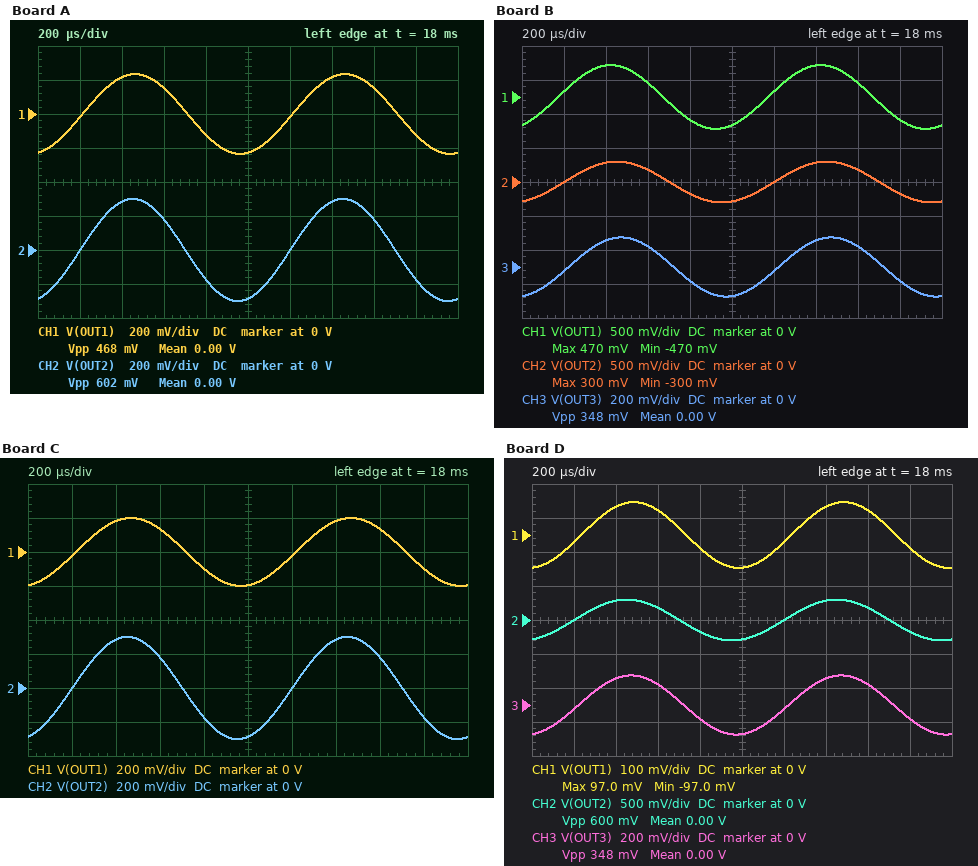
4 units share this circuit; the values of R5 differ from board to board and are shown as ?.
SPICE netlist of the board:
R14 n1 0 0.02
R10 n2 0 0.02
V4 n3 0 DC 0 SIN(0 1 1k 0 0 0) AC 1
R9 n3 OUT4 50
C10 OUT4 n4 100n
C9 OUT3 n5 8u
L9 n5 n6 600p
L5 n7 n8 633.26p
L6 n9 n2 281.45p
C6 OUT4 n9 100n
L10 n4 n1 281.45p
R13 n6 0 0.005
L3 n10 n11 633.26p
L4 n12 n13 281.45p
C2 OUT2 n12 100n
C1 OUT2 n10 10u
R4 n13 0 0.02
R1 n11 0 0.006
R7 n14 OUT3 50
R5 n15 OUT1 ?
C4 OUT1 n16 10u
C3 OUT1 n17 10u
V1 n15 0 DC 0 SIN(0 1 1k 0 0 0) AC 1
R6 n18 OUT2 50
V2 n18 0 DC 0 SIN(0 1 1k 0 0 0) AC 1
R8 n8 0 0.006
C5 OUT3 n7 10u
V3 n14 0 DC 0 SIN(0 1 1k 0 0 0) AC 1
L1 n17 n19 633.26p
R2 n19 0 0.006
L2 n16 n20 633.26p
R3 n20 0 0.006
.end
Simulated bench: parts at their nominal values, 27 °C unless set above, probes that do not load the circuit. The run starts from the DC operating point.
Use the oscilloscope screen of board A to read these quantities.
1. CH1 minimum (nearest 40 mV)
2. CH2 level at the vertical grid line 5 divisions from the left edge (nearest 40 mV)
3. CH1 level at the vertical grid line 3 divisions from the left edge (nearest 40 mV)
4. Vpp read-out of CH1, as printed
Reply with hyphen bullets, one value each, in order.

- -240 mV
- -280 mV
- 160 mV
- 468 mV
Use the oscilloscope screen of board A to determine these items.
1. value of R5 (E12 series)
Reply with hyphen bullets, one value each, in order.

- 33 Ω
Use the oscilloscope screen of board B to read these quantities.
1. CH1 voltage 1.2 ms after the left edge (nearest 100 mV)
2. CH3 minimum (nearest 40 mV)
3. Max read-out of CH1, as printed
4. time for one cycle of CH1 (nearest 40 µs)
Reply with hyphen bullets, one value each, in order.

- 100 mV
- -160 mV
- 470 mV
- 1.00 ms
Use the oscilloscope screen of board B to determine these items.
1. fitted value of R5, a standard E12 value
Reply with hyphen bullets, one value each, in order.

- 15 Ω
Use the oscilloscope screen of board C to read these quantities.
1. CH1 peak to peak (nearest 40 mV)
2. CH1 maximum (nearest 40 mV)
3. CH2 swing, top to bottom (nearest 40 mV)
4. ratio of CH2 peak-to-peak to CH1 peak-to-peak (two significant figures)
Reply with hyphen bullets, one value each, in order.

- 400 mV
- 200 mV
- 600 mV
- 1.5
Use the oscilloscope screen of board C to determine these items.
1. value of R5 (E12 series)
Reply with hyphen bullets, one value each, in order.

- 39 Ω
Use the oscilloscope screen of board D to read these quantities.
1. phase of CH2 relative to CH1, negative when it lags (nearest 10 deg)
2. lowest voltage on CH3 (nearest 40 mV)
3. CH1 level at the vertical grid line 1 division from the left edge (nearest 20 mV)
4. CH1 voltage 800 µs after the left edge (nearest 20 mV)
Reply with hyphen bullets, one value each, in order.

- 10 deg
- -160 mV
- -20 mV
- -40 mV
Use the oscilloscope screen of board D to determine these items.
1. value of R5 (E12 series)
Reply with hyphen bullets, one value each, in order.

- 82 Ω
